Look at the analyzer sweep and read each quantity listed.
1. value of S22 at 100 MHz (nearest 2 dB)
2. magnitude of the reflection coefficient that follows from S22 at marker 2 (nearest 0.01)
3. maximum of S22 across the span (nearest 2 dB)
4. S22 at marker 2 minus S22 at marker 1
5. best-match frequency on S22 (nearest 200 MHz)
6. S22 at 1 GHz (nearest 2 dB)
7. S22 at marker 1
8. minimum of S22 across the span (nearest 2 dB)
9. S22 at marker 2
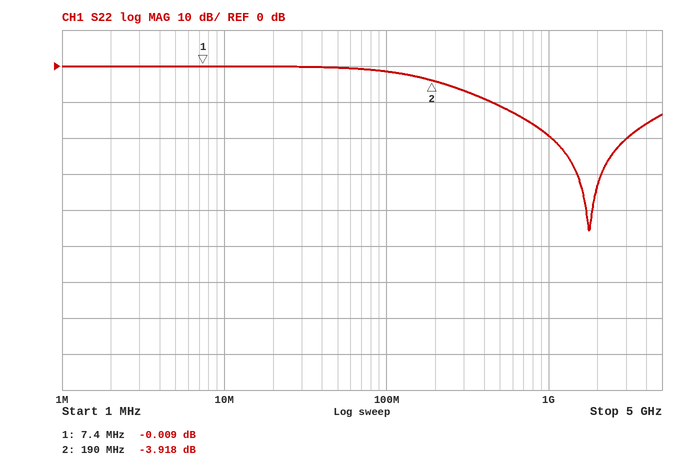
-2 dB
0.64
0 dB
-3.909 dB
1.8 GHz
-20 dB
-0.009 dB
-46 dB
-3.918 dB
